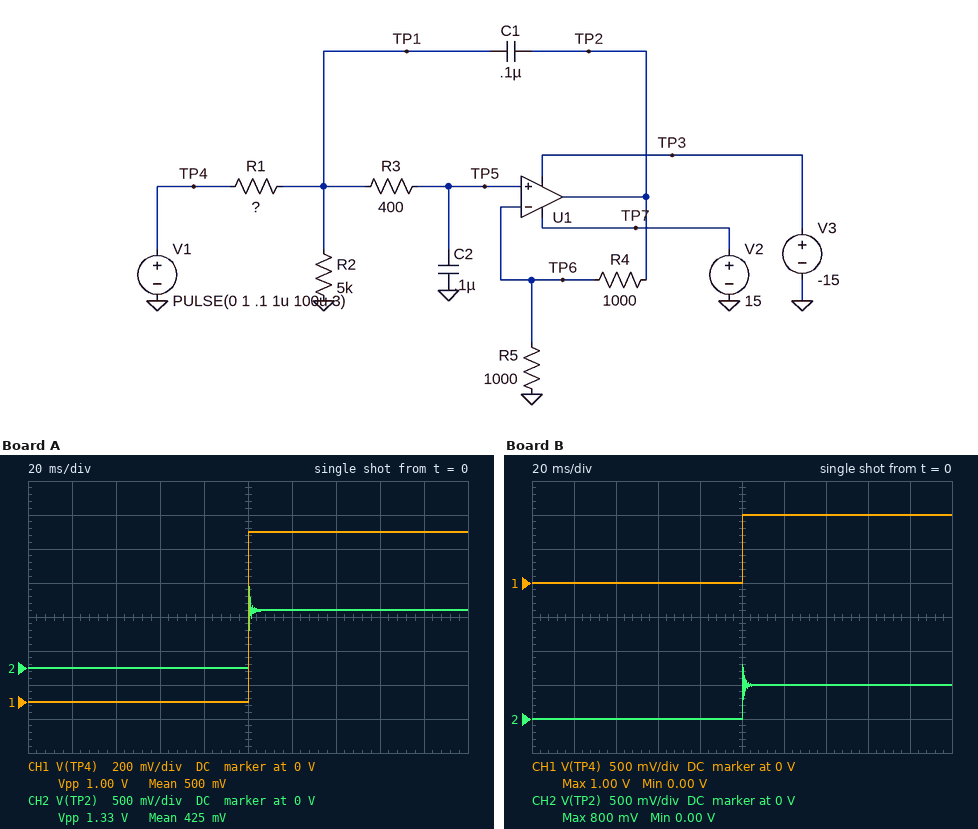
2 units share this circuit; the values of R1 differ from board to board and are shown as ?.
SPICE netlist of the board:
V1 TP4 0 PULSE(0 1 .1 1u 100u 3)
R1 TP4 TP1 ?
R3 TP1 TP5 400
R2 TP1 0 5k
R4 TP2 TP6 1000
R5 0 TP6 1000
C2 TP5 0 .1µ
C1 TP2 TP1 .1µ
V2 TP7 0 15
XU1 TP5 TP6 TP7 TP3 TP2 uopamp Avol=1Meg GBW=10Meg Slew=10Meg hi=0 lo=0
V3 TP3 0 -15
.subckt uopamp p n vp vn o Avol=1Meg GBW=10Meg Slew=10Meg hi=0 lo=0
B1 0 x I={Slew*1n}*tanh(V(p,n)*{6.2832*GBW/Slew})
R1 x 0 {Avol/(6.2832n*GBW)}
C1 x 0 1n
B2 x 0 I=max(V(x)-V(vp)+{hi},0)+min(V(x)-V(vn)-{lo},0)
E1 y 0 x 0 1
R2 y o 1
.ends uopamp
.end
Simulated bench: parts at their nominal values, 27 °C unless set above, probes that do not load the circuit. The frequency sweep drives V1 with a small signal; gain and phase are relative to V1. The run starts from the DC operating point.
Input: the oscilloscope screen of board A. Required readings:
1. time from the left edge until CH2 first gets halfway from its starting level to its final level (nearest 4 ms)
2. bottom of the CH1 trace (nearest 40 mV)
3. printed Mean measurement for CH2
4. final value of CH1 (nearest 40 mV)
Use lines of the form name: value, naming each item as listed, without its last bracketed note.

time from the left edge until CH2 first gets halfway from its starting level to its final level: 100 ms
bottom of the CH1 trace: 0 V
printed Mean measurement for CH2: 425 mV
final value of CH1: 1.00 V
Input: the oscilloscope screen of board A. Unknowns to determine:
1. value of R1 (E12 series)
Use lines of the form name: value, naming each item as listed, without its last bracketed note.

value of R1: 6.8 kΩ
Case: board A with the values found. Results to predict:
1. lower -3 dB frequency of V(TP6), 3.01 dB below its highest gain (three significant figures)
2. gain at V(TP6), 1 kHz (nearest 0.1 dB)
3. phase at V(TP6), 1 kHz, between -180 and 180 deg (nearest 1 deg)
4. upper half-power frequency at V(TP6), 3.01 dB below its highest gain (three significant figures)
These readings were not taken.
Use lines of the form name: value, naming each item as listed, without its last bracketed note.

lower -3 dB frequency of V(TP6), 3.01 dB below its highest gain: 1.11 kHz
gain at V(TP6), 1 kHz: -3.0 dB
phase at V(TP6), 1 kHz, between -180 and 180 deg: -25 deg
upper half-power frequency at V(TP6), 3.01 dB below its highest gain: 1.69 kHz
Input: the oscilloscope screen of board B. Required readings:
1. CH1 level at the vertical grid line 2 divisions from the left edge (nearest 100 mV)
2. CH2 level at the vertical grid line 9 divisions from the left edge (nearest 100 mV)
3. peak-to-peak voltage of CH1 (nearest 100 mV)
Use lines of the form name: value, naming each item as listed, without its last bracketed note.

CH1 level at the vertical grid line 2 divisions from the left edge: 0 V
CH2 level at the vertical grid line 9 divisions from the left edge: 500 mV
peak-to-peak voltage of CH1: 1.0 V
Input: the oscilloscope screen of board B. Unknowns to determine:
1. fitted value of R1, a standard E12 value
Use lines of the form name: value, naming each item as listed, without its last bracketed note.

fitted value of R1, a standard E12 value: 15 kΩ
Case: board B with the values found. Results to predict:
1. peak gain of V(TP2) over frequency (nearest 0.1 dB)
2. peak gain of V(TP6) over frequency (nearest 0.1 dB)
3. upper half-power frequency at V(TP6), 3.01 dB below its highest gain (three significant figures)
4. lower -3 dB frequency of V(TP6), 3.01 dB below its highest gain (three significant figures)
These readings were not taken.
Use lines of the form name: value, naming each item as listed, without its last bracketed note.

peak gain of V(TP2) over frequency: 3.8 dB
peak gain of V(TP6) over frequency: -2.2 dB
upper half-power frequency at V(TP6), 3.01 dB below its highest gain: 1.46 kHz
lower -3 dB frequency of V(TP6), 3.01 dB below its highest gain: 1.03 kHz
